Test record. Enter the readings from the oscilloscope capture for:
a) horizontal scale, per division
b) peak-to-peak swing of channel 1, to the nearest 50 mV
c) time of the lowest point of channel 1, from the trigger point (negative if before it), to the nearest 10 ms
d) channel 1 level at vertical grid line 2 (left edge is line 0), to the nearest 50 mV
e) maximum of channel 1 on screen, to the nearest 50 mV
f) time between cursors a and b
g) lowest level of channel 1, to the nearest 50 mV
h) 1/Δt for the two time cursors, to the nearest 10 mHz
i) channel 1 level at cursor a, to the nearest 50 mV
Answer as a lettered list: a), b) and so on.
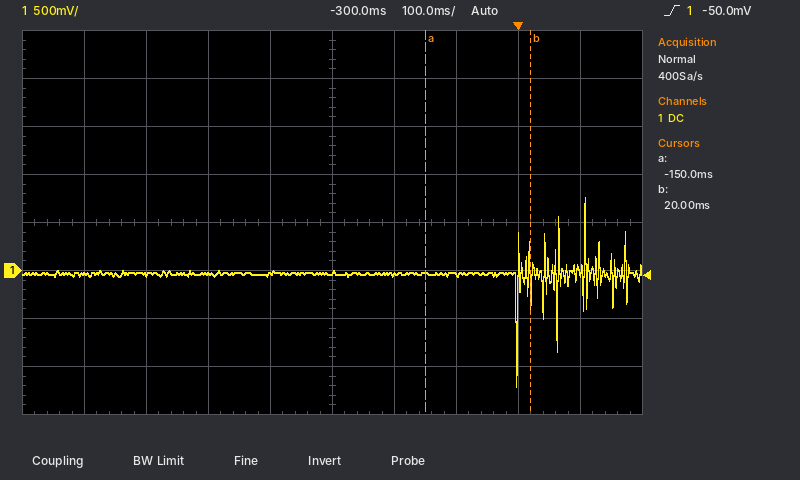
a) 100 ms
b) 1.95 V
c) 0 ms
d) -50 mV
e) 750 mV
f) 170 ms
g) -1.20 V
h) 5.88 Hz
i) -50 mV
